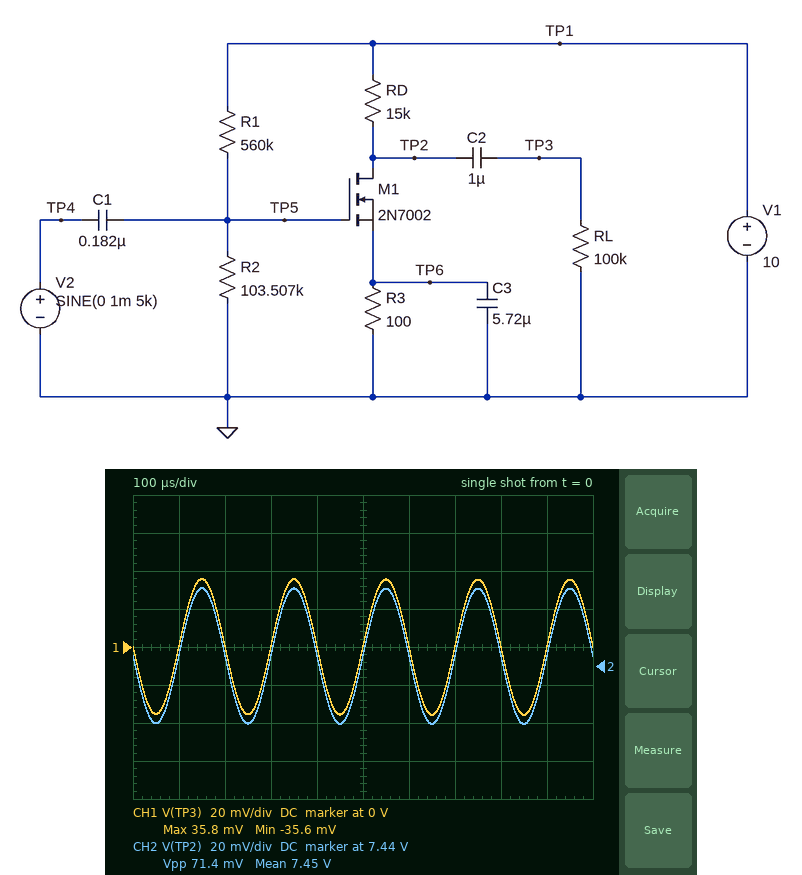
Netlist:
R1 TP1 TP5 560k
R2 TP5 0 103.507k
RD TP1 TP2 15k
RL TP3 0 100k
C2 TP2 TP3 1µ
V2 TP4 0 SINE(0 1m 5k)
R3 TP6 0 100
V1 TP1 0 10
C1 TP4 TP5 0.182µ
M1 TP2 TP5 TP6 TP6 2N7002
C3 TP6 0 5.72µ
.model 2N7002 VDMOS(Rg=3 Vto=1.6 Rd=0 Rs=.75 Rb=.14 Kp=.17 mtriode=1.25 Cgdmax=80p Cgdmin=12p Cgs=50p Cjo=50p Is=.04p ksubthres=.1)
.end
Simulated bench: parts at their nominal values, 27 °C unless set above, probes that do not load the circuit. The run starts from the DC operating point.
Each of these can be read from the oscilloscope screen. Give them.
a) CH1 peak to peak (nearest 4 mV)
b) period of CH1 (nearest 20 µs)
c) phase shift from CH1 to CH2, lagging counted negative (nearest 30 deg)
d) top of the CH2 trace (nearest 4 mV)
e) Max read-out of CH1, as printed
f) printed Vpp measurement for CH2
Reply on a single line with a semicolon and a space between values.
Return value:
72 mV; 200 µs; 0 deg; 7.480 V; 35.8 mV; 71.4 mV
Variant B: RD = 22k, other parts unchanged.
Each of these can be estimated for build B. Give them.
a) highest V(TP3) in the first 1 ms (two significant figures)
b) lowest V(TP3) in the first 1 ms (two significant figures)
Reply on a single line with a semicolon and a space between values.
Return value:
49 mV; -49 mV
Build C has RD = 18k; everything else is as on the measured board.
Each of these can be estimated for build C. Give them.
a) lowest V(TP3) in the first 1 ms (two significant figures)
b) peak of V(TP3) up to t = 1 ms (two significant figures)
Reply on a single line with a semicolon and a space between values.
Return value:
-42 mV; 42 mV
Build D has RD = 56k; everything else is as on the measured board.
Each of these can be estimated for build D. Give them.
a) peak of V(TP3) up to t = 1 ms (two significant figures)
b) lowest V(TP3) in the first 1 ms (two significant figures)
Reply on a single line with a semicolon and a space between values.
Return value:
94 mV; -94 mV
